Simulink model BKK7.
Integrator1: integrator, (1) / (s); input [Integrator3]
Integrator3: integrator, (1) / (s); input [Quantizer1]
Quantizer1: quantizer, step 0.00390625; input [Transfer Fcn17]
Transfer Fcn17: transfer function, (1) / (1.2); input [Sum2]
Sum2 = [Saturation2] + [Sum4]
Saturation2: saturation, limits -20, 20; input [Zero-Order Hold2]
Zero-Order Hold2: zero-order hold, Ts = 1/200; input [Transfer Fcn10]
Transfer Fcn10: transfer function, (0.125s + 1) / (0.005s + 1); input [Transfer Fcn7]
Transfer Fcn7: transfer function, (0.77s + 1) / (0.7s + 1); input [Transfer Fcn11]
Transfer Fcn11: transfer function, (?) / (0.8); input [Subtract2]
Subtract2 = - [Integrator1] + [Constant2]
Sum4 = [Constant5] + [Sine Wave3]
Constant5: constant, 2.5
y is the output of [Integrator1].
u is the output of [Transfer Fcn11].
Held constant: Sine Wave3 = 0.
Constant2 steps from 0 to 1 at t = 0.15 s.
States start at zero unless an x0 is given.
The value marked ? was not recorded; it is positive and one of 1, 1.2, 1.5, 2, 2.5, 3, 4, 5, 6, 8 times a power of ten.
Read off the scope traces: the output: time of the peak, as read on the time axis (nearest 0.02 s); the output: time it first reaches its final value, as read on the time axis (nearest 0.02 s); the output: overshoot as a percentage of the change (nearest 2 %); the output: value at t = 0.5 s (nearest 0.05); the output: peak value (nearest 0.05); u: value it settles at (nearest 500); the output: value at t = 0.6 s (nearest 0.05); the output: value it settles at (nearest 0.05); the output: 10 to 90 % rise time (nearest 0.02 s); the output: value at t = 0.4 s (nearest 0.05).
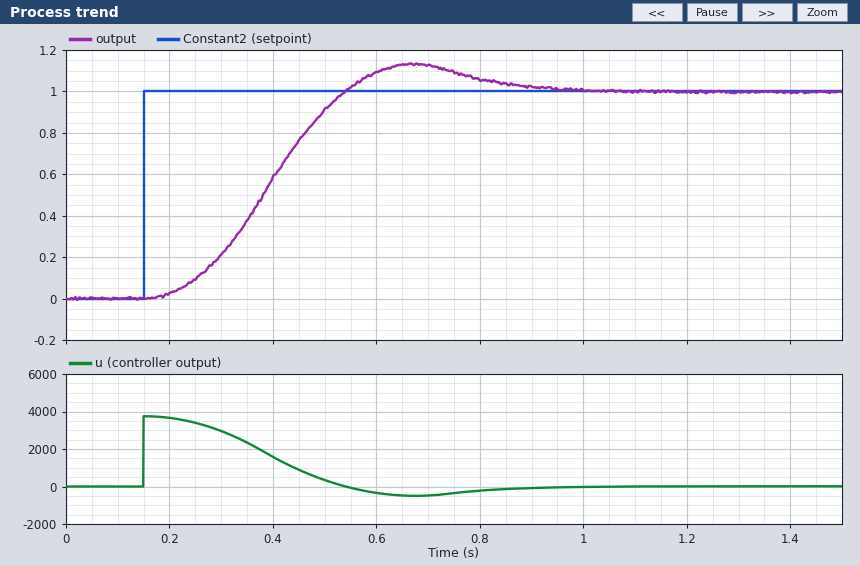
0.68 s
0.54 s
14 %
0.90
1.15
0
1.10
1.00
0.24 s
0.60
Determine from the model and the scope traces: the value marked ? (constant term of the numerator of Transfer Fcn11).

3000
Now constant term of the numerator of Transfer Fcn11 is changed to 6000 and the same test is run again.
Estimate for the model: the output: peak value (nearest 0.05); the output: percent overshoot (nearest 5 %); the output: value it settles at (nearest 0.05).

1.10
10 %
1.00
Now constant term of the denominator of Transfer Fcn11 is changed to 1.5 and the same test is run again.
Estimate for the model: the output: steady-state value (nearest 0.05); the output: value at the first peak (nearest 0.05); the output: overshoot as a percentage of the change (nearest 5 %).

1.00
1.10
10 %
